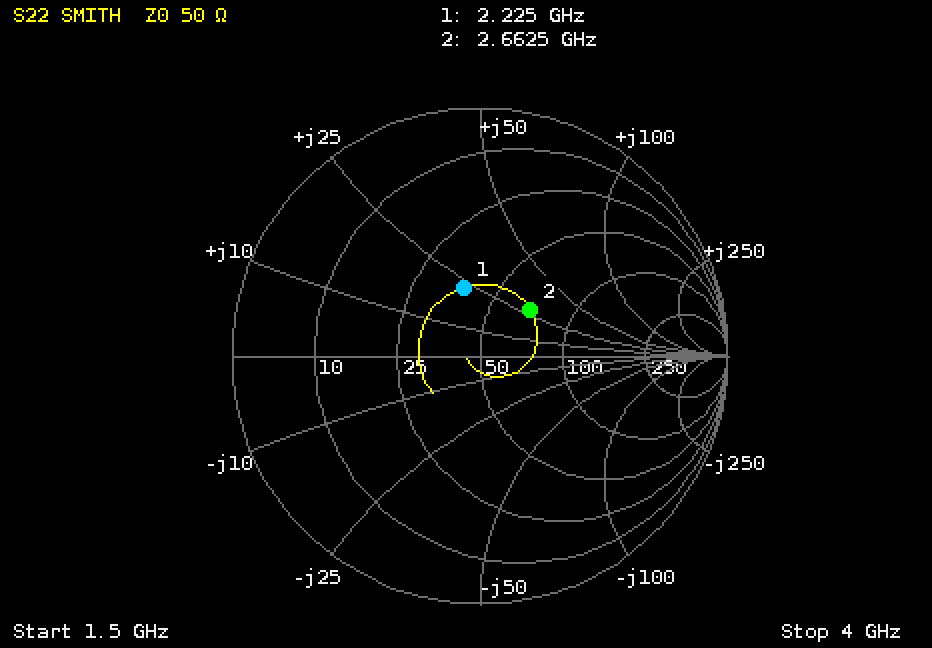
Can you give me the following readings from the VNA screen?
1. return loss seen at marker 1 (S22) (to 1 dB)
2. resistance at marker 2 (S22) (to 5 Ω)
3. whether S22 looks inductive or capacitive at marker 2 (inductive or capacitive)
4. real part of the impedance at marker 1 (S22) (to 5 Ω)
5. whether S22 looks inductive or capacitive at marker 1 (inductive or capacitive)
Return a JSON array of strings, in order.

["11 dB", "70 Ω", "inductive", "40 Ω", "inductive"]
